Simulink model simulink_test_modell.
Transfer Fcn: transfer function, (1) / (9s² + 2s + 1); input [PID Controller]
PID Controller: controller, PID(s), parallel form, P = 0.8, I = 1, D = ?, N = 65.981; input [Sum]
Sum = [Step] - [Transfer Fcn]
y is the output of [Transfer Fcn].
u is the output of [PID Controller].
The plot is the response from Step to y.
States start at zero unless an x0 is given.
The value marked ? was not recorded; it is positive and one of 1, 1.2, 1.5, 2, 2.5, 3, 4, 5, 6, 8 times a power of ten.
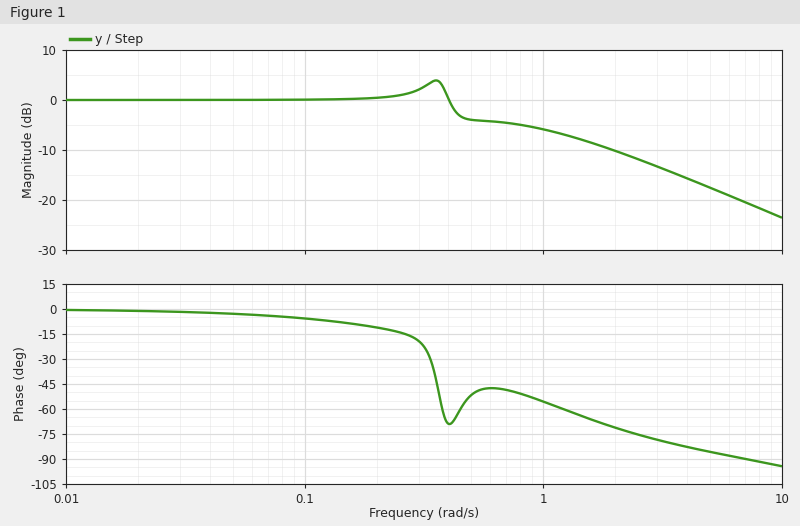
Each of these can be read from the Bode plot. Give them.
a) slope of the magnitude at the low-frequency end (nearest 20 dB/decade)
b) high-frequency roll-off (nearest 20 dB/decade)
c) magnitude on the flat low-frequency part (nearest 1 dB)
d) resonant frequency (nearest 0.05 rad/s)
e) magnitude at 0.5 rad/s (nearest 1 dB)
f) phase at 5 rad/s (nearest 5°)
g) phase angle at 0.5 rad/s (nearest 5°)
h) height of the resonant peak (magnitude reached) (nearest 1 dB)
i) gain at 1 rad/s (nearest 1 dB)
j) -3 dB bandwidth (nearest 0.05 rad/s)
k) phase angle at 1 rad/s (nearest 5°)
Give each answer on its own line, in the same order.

0 dB/decade
-20 dB/decade
0 dB
0.35 rad/s
-4 dB
-85°
-50°
4 dB
-6 dB
0.45 rad/s
-55°
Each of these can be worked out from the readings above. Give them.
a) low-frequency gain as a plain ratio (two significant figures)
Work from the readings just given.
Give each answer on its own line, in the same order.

1.0
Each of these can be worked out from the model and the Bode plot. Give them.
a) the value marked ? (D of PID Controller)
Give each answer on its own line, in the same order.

6
